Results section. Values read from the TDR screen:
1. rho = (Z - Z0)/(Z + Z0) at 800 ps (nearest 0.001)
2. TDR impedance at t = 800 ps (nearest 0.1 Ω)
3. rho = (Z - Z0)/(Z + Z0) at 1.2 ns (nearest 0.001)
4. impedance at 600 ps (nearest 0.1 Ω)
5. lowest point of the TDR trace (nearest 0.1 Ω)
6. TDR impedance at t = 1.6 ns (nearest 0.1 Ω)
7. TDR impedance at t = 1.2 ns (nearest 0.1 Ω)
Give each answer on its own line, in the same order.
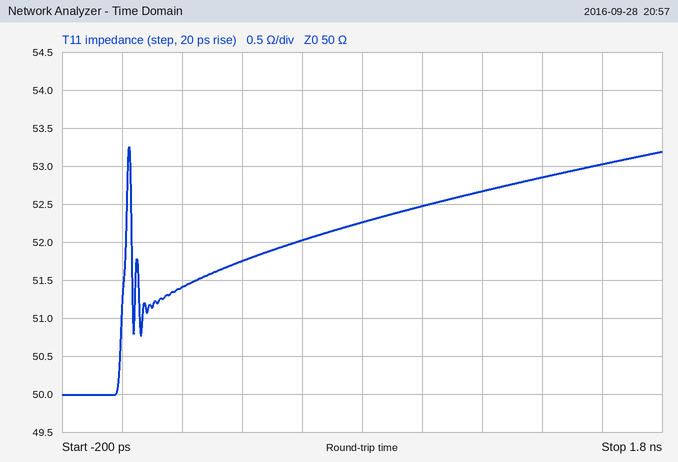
+0.022
52.3 Ω
+0.026
52.0 Ω
50.0 Ω
53.0 Ω
52.7 Ω
